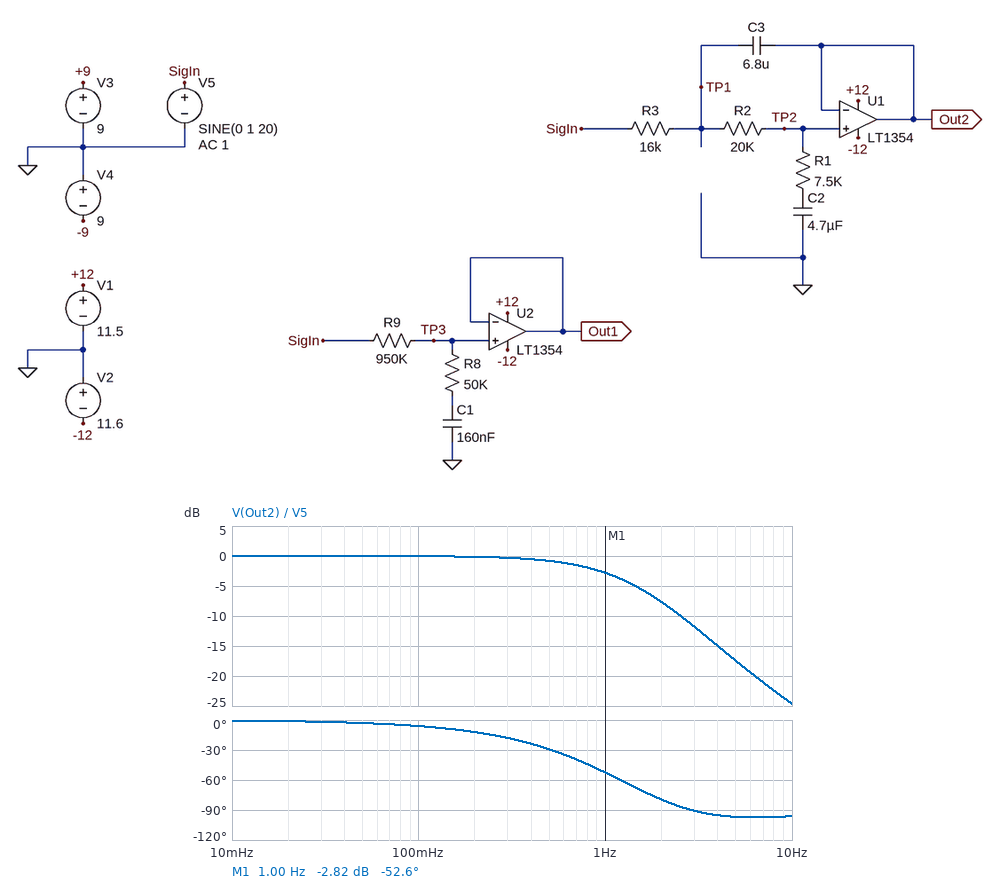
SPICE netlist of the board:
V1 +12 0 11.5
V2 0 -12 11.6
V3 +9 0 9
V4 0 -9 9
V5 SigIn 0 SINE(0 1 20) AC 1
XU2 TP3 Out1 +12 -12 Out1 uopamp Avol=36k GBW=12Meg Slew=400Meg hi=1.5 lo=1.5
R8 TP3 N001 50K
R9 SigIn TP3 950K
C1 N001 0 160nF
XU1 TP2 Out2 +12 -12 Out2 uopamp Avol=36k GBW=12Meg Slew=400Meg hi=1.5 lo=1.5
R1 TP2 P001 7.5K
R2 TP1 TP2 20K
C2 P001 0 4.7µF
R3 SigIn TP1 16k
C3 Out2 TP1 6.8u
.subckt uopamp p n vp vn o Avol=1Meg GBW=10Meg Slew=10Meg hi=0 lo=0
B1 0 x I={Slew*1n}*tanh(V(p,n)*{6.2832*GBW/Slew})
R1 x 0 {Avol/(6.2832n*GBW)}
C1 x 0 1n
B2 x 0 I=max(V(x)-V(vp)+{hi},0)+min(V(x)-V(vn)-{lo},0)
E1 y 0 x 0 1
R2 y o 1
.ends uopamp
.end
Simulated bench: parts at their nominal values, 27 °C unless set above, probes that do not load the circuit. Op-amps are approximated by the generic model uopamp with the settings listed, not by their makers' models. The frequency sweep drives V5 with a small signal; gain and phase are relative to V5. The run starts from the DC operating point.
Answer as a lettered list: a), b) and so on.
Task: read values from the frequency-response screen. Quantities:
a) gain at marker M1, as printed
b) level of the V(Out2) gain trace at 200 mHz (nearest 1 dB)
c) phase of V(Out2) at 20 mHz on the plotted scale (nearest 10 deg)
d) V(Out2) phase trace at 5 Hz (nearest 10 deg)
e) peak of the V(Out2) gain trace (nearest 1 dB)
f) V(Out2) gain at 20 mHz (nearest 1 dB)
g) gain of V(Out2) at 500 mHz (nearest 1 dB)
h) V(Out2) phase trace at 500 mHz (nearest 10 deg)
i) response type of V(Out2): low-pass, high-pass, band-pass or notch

a) -2.82 dB
b) 0 dB
c) 0 deg
d) -100 deg
e) 0 dB
f) 0 dB
g) -1 dB
h) -30 deg
i) low-pass
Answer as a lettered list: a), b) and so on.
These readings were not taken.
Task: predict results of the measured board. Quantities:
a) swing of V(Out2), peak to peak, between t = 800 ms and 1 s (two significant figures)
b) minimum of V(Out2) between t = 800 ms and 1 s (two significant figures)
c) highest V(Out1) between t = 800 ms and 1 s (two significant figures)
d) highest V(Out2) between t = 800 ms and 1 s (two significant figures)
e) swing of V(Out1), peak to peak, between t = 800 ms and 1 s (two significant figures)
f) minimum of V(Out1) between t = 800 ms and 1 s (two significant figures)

a) 56 mV
b) -28 mV
c) 71 mV
d) 28 mV
e) 140 mV
f) -70 mV
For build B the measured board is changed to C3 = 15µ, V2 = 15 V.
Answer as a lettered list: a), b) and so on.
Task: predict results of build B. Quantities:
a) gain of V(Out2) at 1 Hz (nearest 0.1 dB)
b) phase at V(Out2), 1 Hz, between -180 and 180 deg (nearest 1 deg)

a) -2.0 dB
b) -73 deg
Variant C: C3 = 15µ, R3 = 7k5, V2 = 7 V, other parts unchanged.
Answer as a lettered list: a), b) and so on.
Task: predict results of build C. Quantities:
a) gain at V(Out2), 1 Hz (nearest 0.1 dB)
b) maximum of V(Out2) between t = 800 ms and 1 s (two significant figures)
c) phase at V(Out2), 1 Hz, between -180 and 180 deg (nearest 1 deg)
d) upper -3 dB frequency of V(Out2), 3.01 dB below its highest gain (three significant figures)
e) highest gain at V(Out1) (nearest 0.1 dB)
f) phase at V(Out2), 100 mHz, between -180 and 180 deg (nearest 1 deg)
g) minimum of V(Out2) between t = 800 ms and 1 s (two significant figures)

a) -1.3 dB
b) 27 mV
c) -48 deg
d) 1.43 Hz
e) 0 dB
f) -5 deg
g) -27 mV
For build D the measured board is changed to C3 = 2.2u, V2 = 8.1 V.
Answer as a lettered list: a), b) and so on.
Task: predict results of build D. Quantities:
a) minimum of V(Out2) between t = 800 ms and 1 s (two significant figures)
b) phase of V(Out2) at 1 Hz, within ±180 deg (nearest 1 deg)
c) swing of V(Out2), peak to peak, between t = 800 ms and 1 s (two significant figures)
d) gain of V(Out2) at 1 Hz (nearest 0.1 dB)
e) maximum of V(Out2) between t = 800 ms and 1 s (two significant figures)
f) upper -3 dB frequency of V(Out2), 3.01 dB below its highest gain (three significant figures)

a) -79 mV
b) -43 deg
c) 160 mV
d) -3.6 dB
e) 80 mV
f) 876 mHz
